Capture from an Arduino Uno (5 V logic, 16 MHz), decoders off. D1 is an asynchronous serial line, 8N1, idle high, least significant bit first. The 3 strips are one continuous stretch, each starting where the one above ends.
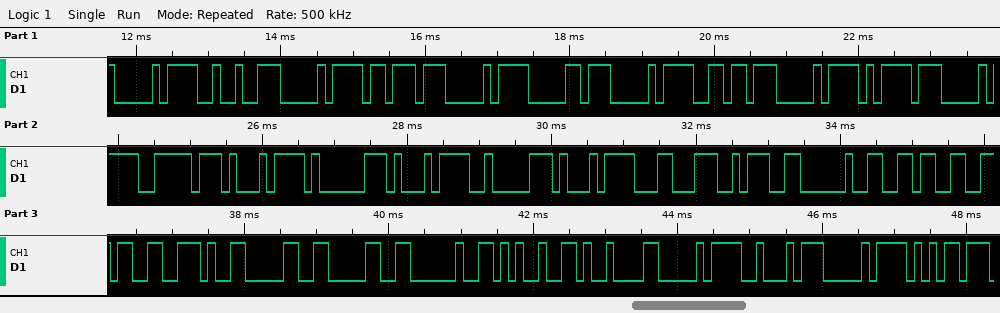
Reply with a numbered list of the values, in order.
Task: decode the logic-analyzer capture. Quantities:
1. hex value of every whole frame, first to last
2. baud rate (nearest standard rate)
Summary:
1. D0 92 D0 BB D0 B0 D0 B6 D0 BD D0 BE D1 81 D1 82 D1 8C 3A 20 36 36 2E 30 30 20 25 09 D0 A2 D0 B5
2. 9600 baud
